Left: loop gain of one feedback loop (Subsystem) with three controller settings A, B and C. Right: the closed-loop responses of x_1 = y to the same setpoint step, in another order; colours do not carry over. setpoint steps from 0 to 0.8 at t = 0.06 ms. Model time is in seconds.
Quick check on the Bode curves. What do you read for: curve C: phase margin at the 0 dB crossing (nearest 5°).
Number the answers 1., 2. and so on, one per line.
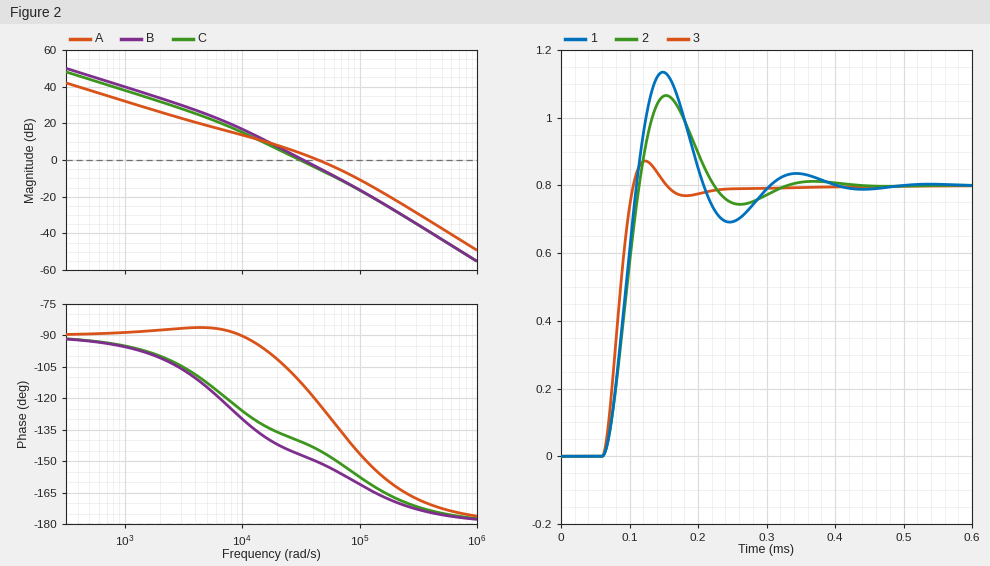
1. 40°
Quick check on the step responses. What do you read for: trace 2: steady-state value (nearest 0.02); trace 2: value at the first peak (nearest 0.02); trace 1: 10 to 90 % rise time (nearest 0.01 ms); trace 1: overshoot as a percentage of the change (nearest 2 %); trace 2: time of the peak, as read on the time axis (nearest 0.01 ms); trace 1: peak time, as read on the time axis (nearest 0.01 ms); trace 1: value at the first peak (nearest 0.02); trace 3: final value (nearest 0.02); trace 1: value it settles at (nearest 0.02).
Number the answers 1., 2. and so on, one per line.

1. 0.80
2. 1.06
3. 0.03 ms
4. 42 %
5. 0.15 ms
6. 0.15 ms
7. 1.14
8. 0.80
9. 0.80
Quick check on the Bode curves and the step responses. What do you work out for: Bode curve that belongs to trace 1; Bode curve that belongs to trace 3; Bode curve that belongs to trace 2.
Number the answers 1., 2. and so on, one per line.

1. B
2. A
3. C
